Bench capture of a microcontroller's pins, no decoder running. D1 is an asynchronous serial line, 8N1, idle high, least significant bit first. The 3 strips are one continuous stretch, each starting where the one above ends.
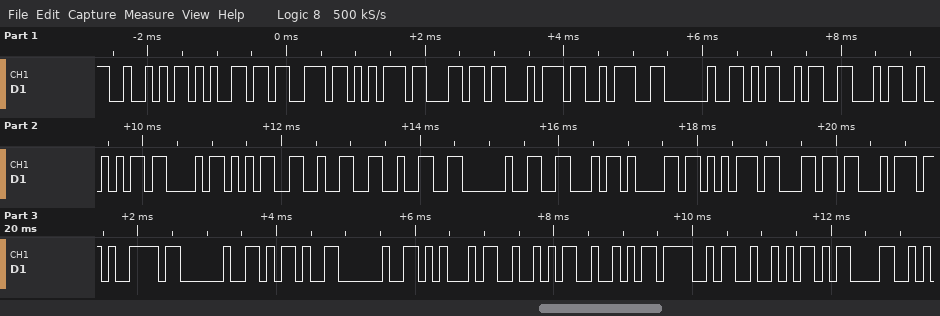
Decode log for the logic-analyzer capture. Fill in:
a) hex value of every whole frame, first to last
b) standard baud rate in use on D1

0x52 0x65 0x73 0x75 0x6C 0x74 0x3A 0x20 0x4D 0x46 0x52 0x43 0x35 0x32 0x32 0x20 0x46 0x61 0x75 0x6C 0x74 0x79 0x20 0x2D 0x20 0x45 0x52 0x52 0x4F 0x52 0x0D
9600 baud
